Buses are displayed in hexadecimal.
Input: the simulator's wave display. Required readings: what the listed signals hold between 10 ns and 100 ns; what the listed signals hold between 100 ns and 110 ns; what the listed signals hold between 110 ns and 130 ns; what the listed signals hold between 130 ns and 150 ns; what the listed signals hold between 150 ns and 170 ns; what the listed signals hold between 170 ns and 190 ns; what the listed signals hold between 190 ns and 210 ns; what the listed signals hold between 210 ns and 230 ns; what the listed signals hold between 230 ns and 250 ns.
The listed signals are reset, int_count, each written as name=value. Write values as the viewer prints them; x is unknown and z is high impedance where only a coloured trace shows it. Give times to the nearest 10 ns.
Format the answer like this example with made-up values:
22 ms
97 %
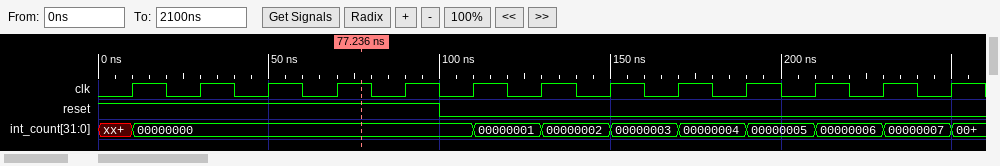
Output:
reset=1, int_count=00000000
reset=0, int_count=00000000
reset=0, int_count=00000001
reset=0, int_count=00000002
reset=0, int_count=00000003
reset=0, int_count=00000004
reset=0, int_count=00000005
reset=0, int_count=00000006
reset=0, int_count=00000007
